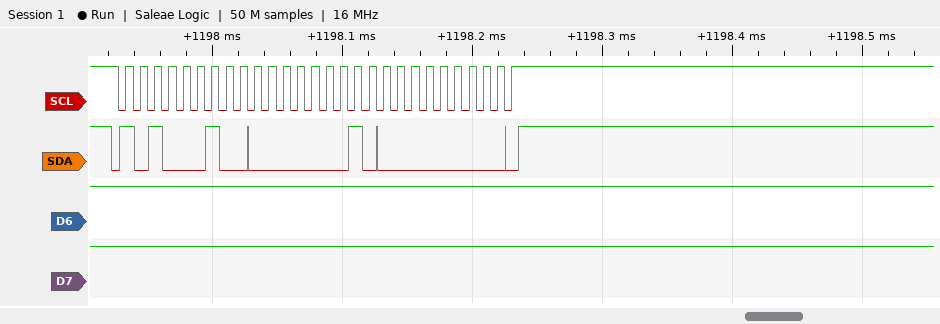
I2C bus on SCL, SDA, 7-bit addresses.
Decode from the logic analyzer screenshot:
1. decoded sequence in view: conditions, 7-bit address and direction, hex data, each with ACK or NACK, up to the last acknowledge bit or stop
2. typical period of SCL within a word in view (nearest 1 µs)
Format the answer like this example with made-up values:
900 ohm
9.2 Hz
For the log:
start, address 51 write ACK, 01 ACK, 00 ACK, stop
11 µs
